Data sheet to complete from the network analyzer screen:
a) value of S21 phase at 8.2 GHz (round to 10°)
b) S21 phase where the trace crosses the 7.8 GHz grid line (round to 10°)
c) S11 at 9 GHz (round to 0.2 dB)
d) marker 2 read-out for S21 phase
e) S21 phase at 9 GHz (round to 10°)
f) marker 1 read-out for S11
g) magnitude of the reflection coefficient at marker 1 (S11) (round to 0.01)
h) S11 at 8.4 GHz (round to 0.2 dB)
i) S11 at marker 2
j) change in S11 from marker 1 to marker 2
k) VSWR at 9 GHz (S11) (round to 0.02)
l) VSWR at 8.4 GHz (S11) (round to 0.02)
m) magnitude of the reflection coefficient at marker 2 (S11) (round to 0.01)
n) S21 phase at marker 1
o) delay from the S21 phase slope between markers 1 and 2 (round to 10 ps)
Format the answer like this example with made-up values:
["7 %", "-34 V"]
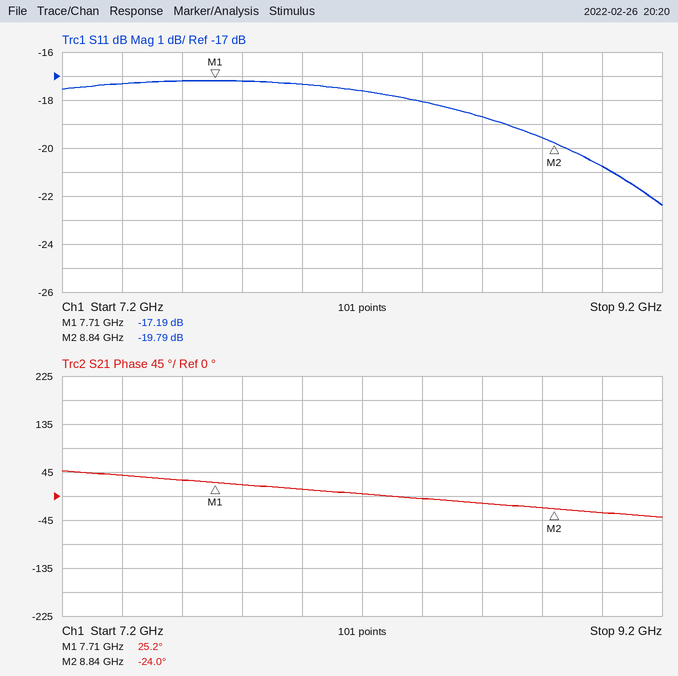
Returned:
["0°", "20°", "-20.8 dB", "-24.0°", "-30°", "-17.19 dB", "0.14", "-18.0 dB", "-19.79 dB", "-2.60 dB", "1.20", "1.28", "0.10", "25.2°", "120 ps"]
